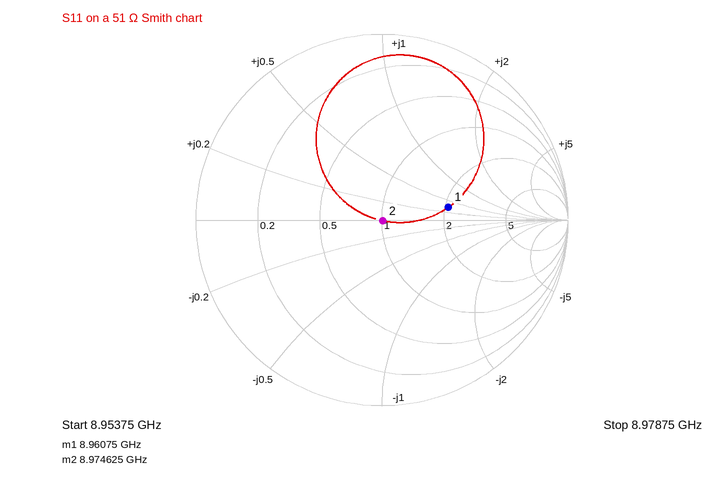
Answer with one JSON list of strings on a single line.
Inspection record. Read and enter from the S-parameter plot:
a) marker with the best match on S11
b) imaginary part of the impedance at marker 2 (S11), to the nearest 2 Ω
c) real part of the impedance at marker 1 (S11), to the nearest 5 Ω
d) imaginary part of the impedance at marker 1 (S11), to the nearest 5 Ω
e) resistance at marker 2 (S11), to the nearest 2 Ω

["marker 2", "0 Ω", "105 Ω", "+15 Ω", "52 Ω"]
